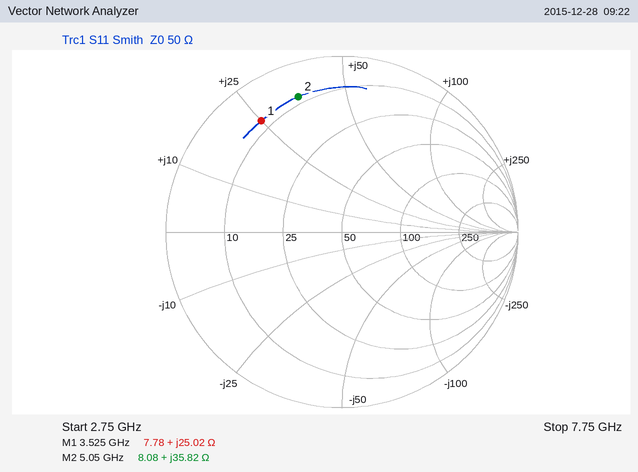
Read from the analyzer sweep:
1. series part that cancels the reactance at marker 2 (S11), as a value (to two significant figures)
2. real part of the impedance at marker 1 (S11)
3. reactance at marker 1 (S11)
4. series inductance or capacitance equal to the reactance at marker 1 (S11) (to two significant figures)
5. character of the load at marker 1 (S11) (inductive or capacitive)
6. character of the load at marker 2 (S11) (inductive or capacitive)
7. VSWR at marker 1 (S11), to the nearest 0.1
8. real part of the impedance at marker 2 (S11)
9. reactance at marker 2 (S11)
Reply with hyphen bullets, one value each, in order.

- 880 fF
- 7.78 Ω
- +25.02 Ω
- 1.1 nH
- inductive
- inductive
- 8.1
- 8.08 Ω
- +35.82 Ω
